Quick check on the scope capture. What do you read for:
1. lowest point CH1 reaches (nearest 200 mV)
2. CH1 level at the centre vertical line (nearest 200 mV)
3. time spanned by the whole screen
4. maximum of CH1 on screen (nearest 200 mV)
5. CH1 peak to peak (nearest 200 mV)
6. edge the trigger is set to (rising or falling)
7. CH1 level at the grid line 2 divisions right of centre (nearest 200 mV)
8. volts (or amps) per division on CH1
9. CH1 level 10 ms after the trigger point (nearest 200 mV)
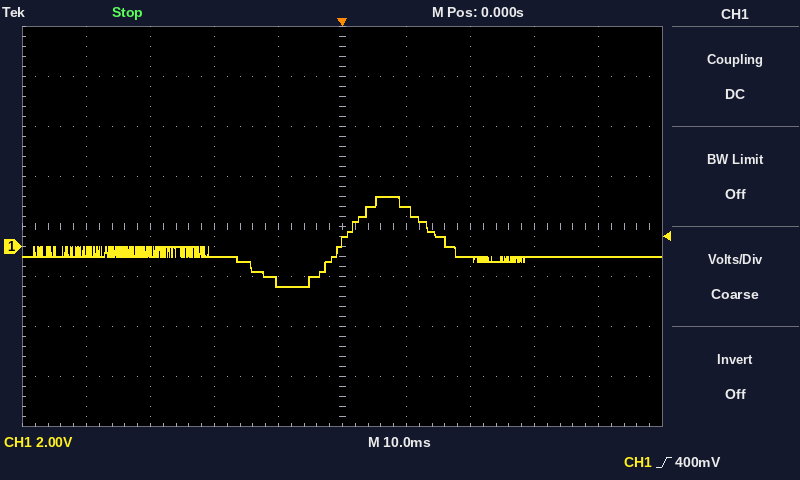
-1.6 V
200 mV
100 ms
2.0 V
3.6 V
rising
-400 mV
2 V
1.6 V
